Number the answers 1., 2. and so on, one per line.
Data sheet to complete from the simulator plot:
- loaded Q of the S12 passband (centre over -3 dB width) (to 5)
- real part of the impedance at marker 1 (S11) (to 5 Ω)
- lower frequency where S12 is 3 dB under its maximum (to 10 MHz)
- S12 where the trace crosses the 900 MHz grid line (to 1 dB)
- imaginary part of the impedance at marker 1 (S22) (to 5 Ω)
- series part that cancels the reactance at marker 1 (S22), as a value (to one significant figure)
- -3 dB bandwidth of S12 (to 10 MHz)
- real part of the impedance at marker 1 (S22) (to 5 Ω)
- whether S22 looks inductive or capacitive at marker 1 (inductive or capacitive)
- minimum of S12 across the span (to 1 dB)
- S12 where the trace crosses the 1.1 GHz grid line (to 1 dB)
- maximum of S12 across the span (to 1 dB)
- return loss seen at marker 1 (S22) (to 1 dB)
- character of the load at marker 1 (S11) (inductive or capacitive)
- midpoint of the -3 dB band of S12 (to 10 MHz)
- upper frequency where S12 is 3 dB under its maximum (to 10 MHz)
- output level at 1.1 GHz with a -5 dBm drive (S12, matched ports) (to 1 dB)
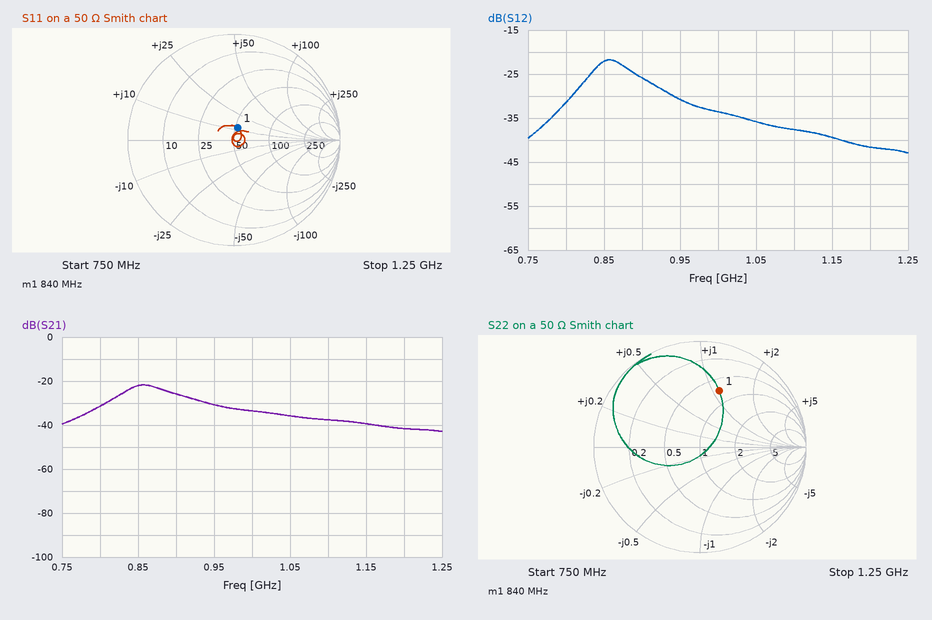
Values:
1. 15
2. 50 Ω
3. 830 MHz
4. -26 dB
5. +55 Ω
6. 3 pF
7. 60 MHz
8. 35 Ω
9. inductive
10. -43 dB
11. -38 dB
12. -22 dB
13. 5 dB
14. inductive
15. 860 MHz
16. 890 MHz
17. -43 dBm
